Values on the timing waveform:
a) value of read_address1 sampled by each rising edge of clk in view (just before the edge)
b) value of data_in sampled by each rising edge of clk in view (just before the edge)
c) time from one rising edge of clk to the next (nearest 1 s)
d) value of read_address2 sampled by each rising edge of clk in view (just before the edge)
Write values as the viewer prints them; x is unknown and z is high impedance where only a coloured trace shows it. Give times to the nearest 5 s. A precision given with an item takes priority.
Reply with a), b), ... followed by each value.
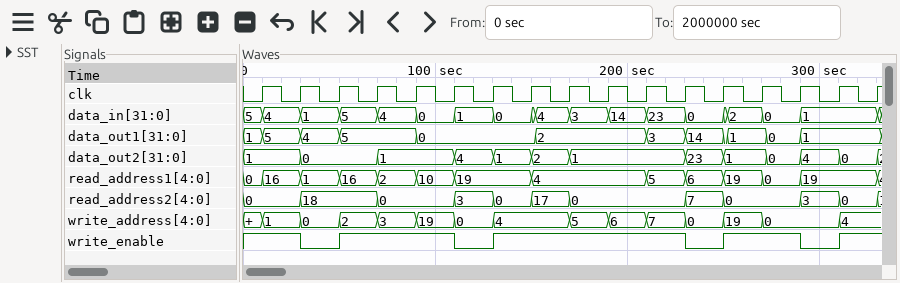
a) 0, 16, 1, 16, 2, 10, 19, 19, 4, 4, 4, 5, 6, 19, 0, 19, 19
b) 5, 4, 1, 5, 4, 0, 1, 0, 4, 3, 14, 23, 0, 2, 0, 1, 1
c) 20 s
d) 0, 0, 18, 18, 0, 0, 3, 0, 17, 0, 0, 0, 7, 0, 0, 3, 0
